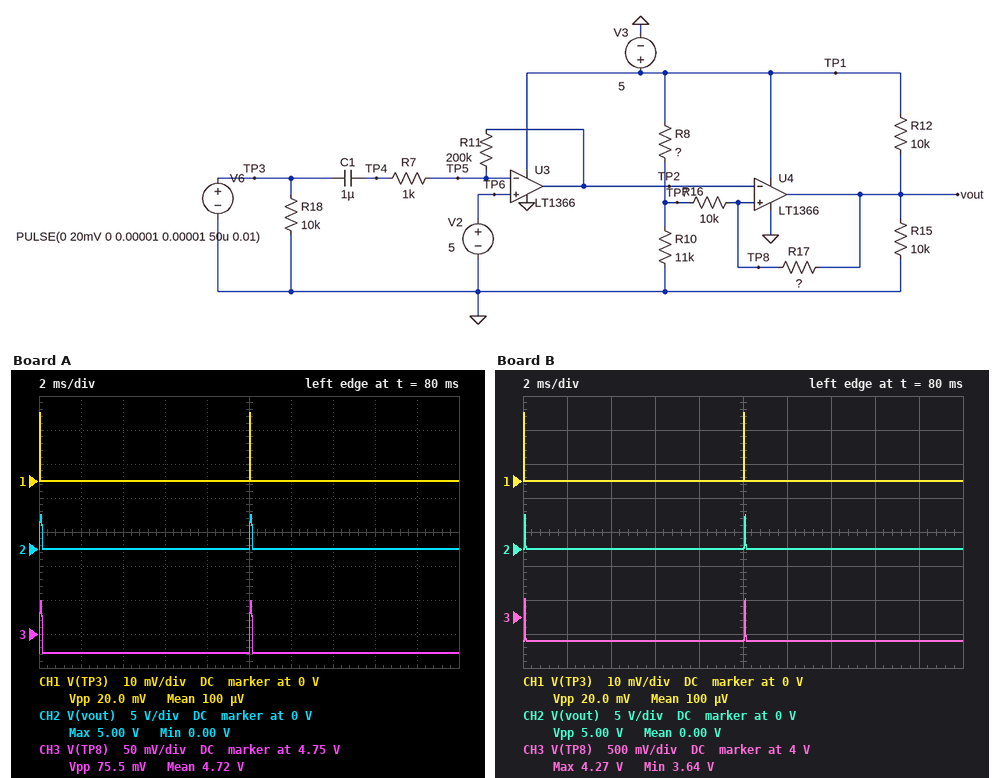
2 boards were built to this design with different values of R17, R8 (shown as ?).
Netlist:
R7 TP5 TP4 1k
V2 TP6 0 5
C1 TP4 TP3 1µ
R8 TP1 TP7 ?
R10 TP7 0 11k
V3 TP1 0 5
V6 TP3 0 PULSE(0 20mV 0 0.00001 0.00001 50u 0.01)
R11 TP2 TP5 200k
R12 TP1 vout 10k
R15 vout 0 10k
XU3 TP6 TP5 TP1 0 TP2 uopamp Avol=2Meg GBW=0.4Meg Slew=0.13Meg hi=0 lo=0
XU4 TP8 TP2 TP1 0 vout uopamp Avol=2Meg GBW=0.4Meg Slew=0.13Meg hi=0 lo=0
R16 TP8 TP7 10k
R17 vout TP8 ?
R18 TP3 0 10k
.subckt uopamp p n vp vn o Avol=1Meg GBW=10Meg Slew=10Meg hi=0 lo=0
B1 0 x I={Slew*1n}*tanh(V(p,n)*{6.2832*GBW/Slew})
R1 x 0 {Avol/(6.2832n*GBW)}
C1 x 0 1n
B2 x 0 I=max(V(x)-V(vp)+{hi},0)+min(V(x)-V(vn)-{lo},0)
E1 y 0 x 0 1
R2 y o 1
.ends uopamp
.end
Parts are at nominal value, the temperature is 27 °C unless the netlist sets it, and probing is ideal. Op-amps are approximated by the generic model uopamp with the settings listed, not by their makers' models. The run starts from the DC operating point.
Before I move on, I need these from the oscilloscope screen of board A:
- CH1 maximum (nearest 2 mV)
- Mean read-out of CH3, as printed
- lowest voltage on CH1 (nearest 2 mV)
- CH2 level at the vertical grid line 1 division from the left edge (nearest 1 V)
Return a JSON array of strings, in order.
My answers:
["20 mV", "4.72 V", "0 V", "0 V"]
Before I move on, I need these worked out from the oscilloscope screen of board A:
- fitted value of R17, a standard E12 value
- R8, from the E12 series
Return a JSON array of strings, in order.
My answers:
["680 kΩ", "470 Ω"]
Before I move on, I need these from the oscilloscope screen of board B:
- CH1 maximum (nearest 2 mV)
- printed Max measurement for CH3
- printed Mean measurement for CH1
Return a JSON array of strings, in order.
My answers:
["20 mV", "4.27 V", "100 µV"]
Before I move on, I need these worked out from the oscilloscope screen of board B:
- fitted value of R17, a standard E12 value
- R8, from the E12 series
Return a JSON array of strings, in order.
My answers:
["82 kΩ", "2.2 kΩ"]
